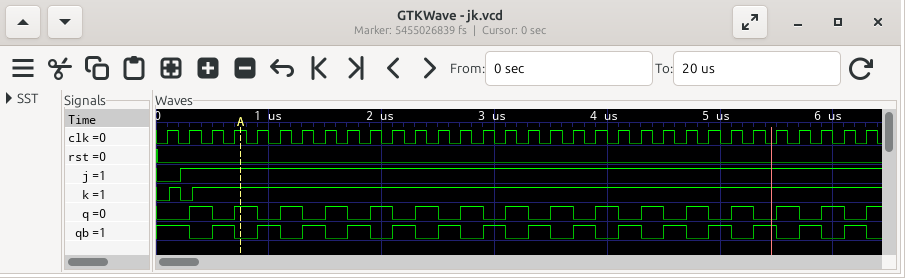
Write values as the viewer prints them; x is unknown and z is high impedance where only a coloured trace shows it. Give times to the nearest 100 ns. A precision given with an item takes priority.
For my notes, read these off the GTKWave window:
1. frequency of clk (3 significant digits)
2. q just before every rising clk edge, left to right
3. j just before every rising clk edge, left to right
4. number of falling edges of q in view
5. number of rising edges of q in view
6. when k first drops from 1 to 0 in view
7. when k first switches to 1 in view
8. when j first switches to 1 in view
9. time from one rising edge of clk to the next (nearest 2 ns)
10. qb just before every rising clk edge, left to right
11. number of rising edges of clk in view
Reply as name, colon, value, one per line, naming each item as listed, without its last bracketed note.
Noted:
frequency of clk: 5.00 MHz
q just before every rising clk edge, left to right: 0 0 1 0 1 0 1 0 1 0 1 0 1 0 1 0 1 0 1 0 1 0 1 0 1 0 1 0 1 0 1 0
j just before every rising clk edge, left to right: 0 1 1 1 1 1 1 1 1 1 1 1 1 1 1 1 1 1 1 1 1 1 1 1 1 1 1 1 1 1 1 1
number of falling edges of q in view: 15
number of rising edges of q in view: 16
when k first drops from 1 to 0 in view: 200 ns
when k first switches to 1 in view: 100 ns
when j first switches to 1 in view: 200 ns
time from one rising edge of clk to the next: 200 ns
qb just before every rising clk edge, left to right: 1 1 0 1 0 1 0 1 0 1 0 1 0 1 0 1 0 1 0 1 0 1 0 1 0 1 0 1 0 1 0 1
number of rising edges of clk in view: 32
